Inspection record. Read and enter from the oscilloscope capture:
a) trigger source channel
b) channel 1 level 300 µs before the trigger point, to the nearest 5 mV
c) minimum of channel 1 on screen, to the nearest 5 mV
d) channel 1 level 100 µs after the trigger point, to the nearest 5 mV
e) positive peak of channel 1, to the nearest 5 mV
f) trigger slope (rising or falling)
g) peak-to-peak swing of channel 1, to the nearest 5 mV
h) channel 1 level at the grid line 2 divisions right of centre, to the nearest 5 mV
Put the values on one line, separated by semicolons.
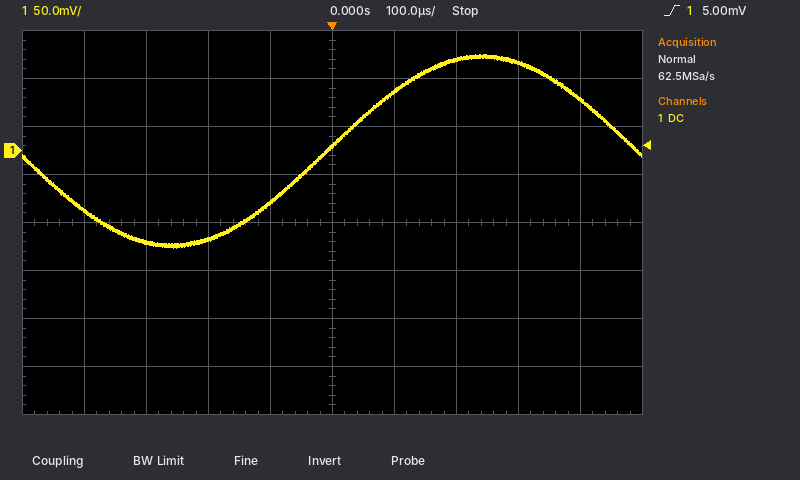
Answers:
channel 1; -95 mV; -100 mV; 60 mV; 100 mV; rising; 200 mV; 95 mV
